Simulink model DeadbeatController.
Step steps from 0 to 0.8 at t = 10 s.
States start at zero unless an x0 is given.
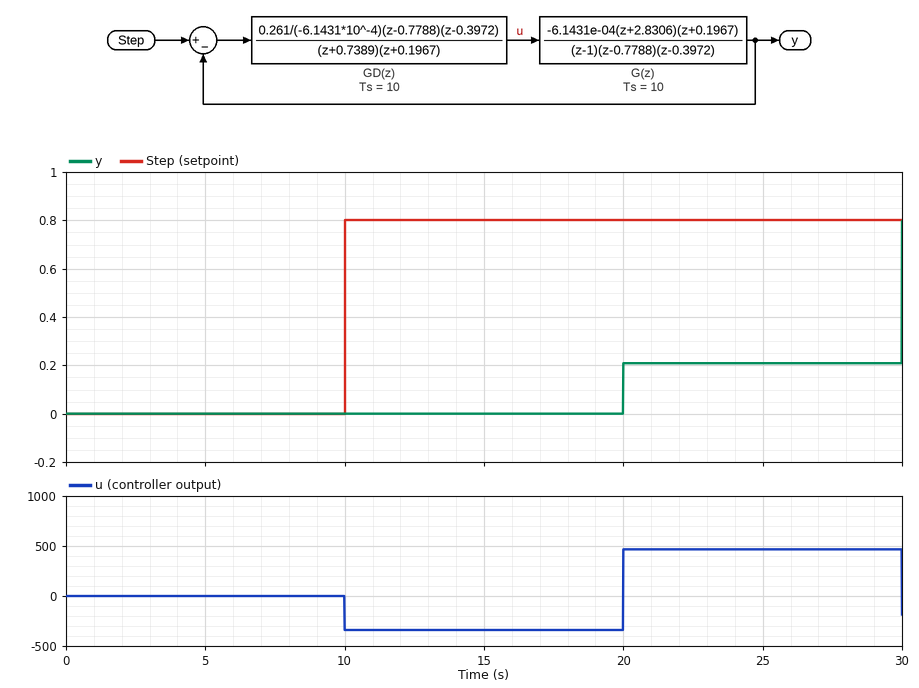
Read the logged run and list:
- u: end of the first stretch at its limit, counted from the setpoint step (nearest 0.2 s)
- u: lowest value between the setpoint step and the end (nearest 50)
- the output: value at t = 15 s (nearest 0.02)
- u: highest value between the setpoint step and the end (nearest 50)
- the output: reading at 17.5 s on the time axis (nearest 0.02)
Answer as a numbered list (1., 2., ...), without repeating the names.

1. 10.0 s
2. -350
3. 0.00
4. 450
5. 0.00
